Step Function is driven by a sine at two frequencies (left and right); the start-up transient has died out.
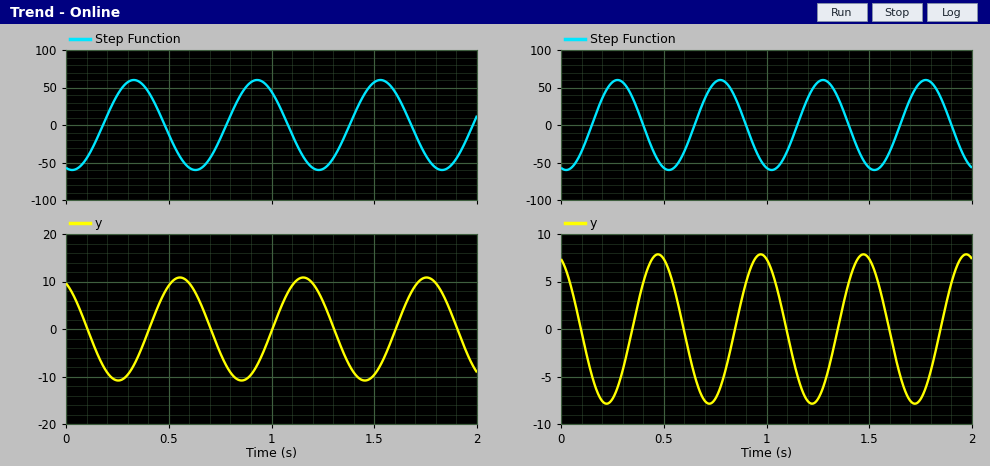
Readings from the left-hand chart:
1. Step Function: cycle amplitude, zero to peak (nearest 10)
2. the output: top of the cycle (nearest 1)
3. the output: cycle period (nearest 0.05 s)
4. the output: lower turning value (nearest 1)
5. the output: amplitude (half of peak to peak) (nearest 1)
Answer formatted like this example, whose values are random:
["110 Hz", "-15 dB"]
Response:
["60", "11", "0.60 s", "-11", "11"]
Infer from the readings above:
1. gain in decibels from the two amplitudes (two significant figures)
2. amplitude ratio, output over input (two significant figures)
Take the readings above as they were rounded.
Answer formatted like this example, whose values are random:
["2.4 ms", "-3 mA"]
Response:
["-15 dB", "0.18"]
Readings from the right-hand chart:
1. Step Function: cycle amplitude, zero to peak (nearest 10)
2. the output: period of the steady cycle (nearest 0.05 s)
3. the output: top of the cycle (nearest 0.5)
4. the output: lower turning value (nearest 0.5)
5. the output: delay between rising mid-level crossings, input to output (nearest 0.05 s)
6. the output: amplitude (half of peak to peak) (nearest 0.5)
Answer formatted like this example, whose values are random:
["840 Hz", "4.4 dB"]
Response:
["60", "0.50 s", "8.0", "-8.0", "0.20 s", "8.0"]
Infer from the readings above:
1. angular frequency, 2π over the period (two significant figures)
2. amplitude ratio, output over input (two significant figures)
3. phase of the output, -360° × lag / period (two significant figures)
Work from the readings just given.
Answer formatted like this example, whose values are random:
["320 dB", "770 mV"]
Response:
["13 rad/s", "0.13", "-140°"]
